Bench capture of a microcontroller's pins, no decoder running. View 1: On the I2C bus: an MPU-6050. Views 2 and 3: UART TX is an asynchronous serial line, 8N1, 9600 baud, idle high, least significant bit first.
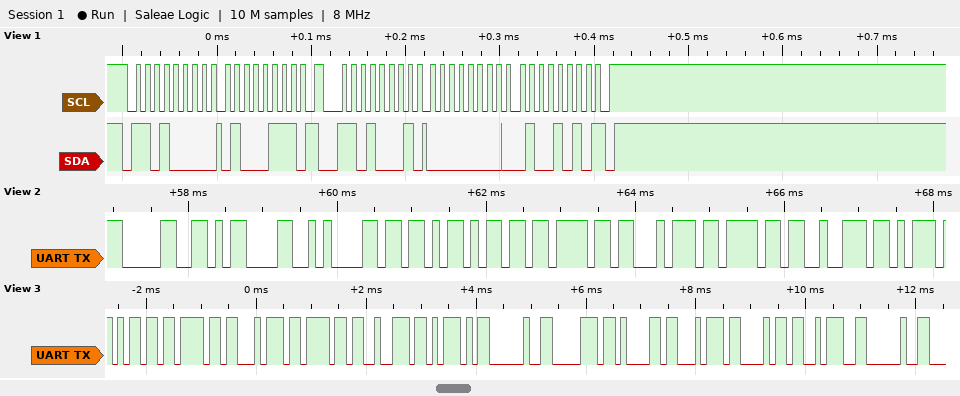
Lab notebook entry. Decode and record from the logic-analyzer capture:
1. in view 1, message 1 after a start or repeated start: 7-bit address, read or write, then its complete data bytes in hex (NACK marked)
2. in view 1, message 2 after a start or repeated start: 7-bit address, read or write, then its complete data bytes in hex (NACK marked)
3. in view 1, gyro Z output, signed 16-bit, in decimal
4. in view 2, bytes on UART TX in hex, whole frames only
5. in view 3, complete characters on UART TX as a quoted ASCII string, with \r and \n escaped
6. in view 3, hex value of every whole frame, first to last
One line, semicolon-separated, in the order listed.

0x68 write: 47; 0x68 read: 00 4A NACK; 74; 0x30 0x0D 0x0A 0x5B 0x6D 0x6F 0x74 0x6F 0x72; "motor] path: "; 6D 6F 74 6F 72 5D 20 70 61 74 68 3A 20
